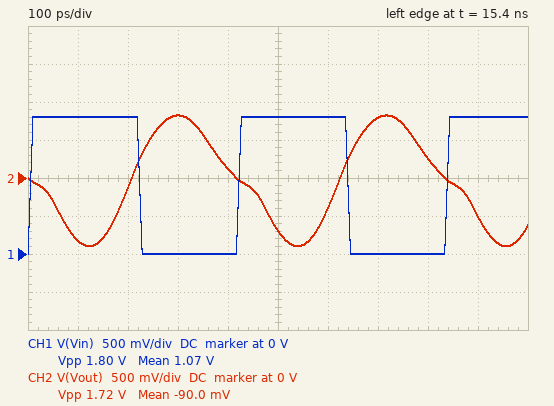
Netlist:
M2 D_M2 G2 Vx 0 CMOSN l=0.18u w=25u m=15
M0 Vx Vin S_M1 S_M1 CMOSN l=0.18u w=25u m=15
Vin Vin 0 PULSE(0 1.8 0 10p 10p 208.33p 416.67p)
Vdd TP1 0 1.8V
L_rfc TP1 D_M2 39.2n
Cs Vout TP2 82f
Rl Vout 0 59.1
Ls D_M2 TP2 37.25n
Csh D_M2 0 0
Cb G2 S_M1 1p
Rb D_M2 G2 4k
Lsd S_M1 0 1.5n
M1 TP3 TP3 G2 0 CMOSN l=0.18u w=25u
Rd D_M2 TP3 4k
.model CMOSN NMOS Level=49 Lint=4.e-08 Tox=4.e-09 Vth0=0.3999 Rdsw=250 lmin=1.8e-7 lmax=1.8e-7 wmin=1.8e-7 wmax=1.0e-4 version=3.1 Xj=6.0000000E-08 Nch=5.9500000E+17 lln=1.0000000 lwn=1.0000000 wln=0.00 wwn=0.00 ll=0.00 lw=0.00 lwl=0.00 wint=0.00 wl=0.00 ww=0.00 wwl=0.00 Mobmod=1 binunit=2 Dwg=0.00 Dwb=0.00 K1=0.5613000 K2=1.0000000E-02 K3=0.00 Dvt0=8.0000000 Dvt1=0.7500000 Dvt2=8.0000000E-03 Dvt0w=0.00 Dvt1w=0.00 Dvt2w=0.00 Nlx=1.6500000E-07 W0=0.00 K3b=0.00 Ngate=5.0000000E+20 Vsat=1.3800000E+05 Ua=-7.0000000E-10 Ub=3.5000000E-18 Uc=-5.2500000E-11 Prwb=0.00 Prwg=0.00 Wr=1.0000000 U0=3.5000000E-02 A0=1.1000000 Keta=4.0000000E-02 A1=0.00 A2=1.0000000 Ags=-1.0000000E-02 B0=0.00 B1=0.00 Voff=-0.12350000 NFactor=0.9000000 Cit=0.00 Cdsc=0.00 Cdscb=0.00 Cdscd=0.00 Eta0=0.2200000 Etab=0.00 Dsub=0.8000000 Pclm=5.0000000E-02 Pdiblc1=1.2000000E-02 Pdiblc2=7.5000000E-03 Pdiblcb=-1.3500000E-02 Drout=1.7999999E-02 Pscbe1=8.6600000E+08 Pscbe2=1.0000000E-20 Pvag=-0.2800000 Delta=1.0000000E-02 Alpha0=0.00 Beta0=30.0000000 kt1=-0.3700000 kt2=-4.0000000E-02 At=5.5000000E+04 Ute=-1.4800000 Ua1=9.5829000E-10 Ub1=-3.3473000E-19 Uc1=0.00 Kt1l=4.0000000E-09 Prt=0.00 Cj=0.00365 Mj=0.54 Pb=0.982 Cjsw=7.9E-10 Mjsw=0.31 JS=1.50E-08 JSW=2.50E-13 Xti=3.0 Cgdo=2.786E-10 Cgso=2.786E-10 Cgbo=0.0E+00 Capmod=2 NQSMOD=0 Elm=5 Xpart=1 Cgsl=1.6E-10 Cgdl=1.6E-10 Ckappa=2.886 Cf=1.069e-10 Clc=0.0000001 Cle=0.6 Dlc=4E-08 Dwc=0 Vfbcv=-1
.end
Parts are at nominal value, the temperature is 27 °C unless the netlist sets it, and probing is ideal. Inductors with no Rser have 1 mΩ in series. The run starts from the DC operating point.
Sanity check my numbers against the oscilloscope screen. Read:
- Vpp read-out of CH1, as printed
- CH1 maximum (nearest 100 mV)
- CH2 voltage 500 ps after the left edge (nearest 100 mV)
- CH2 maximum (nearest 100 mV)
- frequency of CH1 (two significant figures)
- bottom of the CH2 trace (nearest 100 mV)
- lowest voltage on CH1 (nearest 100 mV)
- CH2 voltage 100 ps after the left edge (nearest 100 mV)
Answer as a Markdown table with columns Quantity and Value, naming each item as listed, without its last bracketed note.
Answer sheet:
| Quantity | Value |
|---|---|
| Vpp read-out of CH1, as printed | 1.80 V |
| CH1 maximum | 1.8 V |
| CH2 voltage 500 ps after the left edge | -700 mV |
| CH2 maximum | 800 mV |
| frequency of CH1 | 2.4 GHz |
| bottom of the CH2 trace | -900 mV |
| lowest voltage on CH1 | 0 V |
| CH2 voltage 100 ps after the left edge | -800 mV |
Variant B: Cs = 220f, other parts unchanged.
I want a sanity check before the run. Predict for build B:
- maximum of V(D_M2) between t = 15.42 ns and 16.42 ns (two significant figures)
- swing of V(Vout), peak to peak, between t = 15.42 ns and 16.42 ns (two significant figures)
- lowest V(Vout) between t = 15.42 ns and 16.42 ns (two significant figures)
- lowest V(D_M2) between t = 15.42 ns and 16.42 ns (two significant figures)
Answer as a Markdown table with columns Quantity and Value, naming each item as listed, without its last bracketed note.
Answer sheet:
| Quantity | Value |
|---|---|
| maximum of V(D_M2) between t = 15.42 ns and 16.42 ns | 7.3 V |
| swing of V(Vout), peak to peak, between t = 15.42 ns and 16.42 ns | 1.3 V |
| lowest V(Vout) between t = 15.42 ns and 16.42 ns | -570 mV |
| lowest V(D_M2) between t = 15.42 ns and 16.42 ns | -870 mV |
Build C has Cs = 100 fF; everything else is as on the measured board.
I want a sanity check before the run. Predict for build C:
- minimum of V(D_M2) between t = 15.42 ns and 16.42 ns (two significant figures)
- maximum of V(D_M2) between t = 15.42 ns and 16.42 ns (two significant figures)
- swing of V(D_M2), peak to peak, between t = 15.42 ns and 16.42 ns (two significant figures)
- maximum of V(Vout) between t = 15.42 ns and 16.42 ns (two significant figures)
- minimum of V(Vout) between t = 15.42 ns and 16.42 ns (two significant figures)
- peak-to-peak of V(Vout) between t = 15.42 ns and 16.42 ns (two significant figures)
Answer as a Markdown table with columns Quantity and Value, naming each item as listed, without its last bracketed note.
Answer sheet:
| Quantity | Value |
|---|---|
| minimum of V(D_M2) between t = 15.42 ns and 16.42 ns | -1.6 V |
| maximum of V(D_M2) between t = 15.42 ns and 16.42 ns | 10 V |
| swing of V(D_M2), peak to peak, between t = 15.42 ns and 16.42 ns | 12 V |
| maximum of V(Vout) between t = 15.42 ns and 16.42 ns | 1.7 V |
| minimum of V(Vout) between t = 15.42 ns and 16.42 ns | -1.9 V |
| peak-to-peak of V(Vout) between t = 15.42 ns and 16.42 ns | 3.6 V |
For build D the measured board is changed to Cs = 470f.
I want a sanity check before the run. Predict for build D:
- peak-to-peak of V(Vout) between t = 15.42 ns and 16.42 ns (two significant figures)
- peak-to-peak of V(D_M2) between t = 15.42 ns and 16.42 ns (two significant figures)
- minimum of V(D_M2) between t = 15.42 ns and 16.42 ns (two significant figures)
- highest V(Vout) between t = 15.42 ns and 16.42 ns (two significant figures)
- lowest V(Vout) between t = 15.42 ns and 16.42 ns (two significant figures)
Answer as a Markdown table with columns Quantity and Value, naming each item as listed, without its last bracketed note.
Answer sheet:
| Quantity | Value |
|---|---|
| peak-to-peak of V(Vout) between t = 15.42 ns and 16.42 ns | 820 mV |
| peak-to-peak of V(D_M2) between t = 15.42 ns and 16.42 ns | 8.0 V |
| minimum of V(D_M2) between t = 15.42 ns and 16.42 ns | -1.1 V |
| highest V(Vout) between t = 15.42 ns and 16.42 ns | 420 mV |
| lowest V(Vout) between t = 15.42 ns and 16.42 ns | -390 mV |
